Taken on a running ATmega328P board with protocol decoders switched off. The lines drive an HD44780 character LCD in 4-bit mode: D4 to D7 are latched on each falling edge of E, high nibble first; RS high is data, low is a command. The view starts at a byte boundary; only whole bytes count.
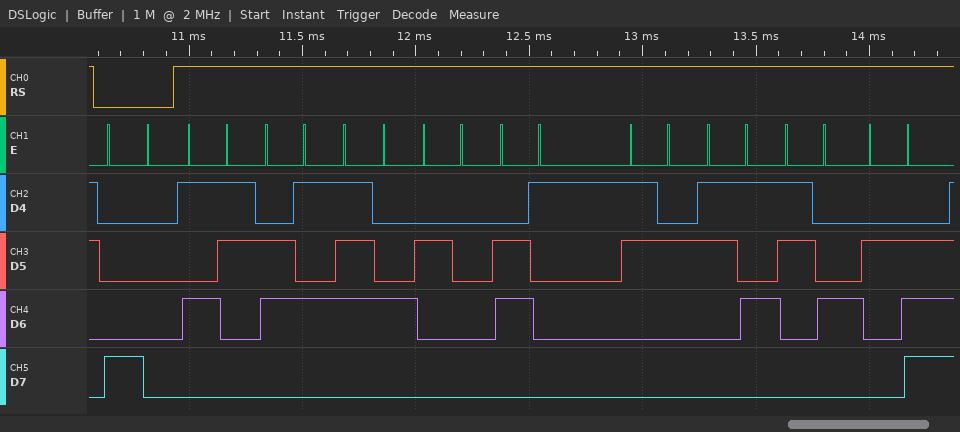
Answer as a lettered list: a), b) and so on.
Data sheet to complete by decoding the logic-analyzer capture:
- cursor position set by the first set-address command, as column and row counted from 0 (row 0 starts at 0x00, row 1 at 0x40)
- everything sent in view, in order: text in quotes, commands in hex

a) column 0, row 0
b) 0x80 "Set a254."
